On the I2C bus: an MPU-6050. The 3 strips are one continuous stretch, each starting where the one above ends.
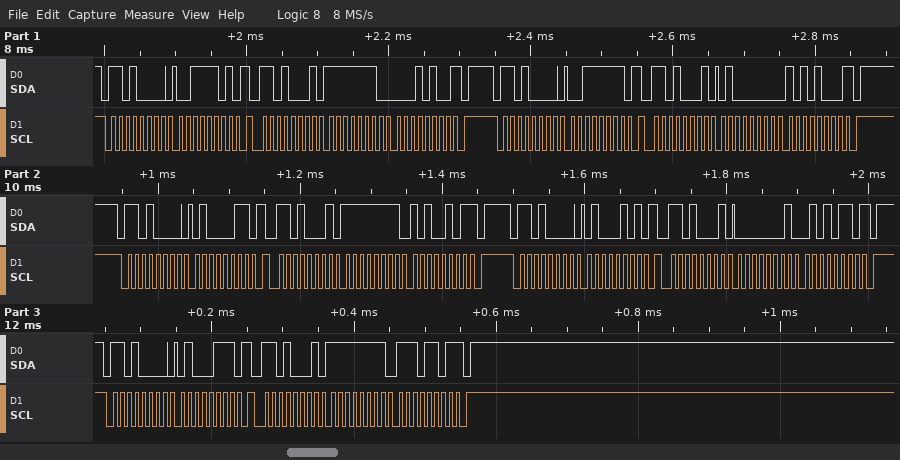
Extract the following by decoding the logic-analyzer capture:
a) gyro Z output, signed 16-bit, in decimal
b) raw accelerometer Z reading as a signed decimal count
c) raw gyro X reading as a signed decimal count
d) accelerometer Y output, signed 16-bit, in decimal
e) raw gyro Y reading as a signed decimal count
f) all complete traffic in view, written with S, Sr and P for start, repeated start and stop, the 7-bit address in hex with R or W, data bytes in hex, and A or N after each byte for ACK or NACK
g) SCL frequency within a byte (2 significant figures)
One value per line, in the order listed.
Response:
-19
16552
-91
-492
342
S 68W A 3D A Sr 68R A FE A 14 N P S 68W A 3F A Sr 68R A 40 A A8 N P S 68W A 43 A Sr 68R A FF A A5 N P S 68W A 45 A Sr 68R A 01 A 56 N P S 68W A 47 A Sr 68R A FF A ED N P
100 kHz
